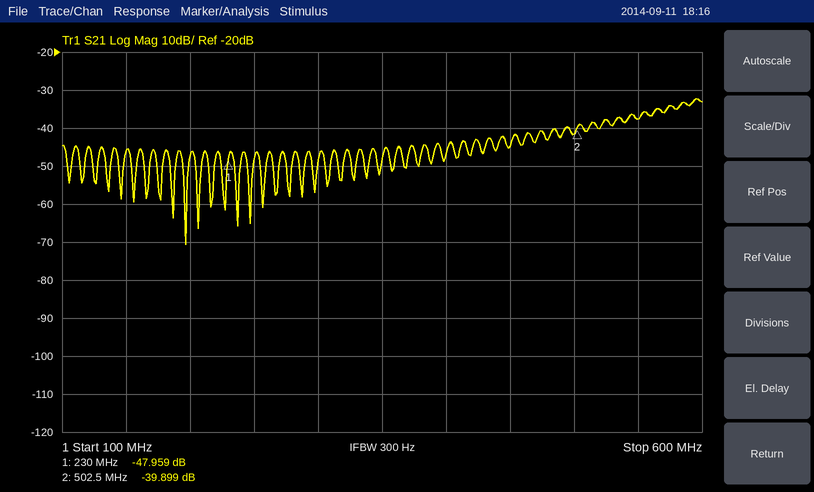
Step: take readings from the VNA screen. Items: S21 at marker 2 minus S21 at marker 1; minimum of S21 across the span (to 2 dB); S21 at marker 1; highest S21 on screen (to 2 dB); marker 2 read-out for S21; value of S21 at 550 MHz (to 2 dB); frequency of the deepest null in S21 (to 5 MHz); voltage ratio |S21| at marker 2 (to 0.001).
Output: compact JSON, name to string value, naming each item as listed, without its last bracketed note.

{"S21 at marker 2 minus S21 at marker 1": "8.060 dB", "minimum of S21 across the span": "-70 dB", "S21 at marker 1": "-47.959 dB", "highest S21 on screen": "-32 dB", "marker 2 read-out for S21": "-39.899 dB", "value of S21 at 550 MHz": "-38 dB", "frequency of the deepest null in S21": "195 MHz", "voltage ratio |S21| at marker 2": "0.010"}
